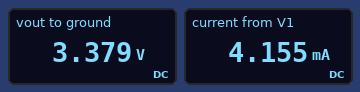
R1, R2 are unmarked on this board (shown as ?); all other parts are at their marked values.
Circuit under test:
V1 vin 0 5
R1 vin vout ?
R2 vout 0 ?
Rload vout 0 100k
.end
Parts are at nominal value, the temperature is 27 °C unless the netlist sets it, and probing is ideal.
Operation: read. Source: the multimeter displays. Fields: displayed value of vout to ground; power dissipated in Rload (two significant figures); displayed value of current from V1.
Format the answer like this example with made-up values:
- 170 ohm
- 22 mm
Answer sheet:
- 3.379 V
- 110 µW
- 4.155 mA
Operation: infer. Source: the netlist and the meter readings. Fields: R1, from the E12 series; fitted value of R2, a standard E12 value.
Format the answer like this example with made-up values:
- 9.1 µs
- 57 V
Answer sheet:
- 390 Ω
- 820 Ω
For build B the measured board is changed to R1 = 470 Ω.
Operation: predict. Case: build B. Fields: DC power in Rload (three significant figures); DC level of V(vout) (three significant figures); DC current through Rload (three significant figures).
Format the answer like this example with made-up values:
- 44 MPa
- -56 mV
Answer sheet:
- 100 µW
- 3.17 V
- 31.7 µA
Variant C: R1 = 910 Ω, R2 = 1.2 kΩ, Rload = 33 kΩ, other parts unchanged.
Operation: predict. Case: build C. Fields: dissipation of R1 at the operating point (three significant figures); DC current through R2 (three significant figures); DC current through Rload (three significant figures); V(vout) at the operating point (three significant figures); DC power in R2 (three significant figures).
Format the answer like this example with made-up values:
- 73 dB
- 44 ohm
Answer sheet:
- 5.32 mW
- 2.33 mA
- 84.8 µA
- 2.80 V
- 6.53 mW
